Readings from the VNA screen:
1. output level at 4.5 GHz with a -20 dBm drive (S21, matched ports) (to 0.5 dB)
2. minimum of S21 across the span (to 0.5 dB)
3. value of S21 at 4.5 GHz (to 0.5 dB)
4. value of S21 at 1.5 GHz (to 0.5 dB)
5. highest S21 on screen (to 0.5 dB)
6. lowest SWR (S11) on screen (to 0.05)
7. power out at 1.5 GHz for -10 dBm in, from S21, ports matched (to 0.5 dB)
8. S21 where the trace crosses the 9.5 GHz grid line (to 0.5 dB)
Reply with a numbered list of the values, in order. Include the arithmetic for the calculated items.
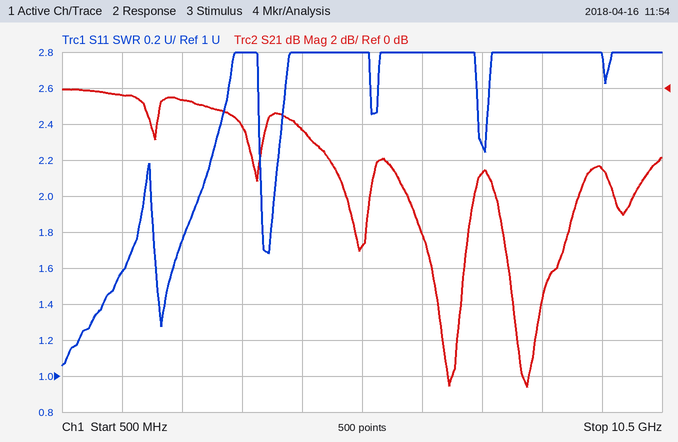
1. -20 dBm + (-2.5 dB) = -22.5 dBm
2. -16.5 dB
3. -2.5 dB
4. -0.5 dB
5. 0.0 dB
6. 1.05
7. -10 dBm + (-0.5 dB) = -10.5 dBm
8. -4.5 dB
